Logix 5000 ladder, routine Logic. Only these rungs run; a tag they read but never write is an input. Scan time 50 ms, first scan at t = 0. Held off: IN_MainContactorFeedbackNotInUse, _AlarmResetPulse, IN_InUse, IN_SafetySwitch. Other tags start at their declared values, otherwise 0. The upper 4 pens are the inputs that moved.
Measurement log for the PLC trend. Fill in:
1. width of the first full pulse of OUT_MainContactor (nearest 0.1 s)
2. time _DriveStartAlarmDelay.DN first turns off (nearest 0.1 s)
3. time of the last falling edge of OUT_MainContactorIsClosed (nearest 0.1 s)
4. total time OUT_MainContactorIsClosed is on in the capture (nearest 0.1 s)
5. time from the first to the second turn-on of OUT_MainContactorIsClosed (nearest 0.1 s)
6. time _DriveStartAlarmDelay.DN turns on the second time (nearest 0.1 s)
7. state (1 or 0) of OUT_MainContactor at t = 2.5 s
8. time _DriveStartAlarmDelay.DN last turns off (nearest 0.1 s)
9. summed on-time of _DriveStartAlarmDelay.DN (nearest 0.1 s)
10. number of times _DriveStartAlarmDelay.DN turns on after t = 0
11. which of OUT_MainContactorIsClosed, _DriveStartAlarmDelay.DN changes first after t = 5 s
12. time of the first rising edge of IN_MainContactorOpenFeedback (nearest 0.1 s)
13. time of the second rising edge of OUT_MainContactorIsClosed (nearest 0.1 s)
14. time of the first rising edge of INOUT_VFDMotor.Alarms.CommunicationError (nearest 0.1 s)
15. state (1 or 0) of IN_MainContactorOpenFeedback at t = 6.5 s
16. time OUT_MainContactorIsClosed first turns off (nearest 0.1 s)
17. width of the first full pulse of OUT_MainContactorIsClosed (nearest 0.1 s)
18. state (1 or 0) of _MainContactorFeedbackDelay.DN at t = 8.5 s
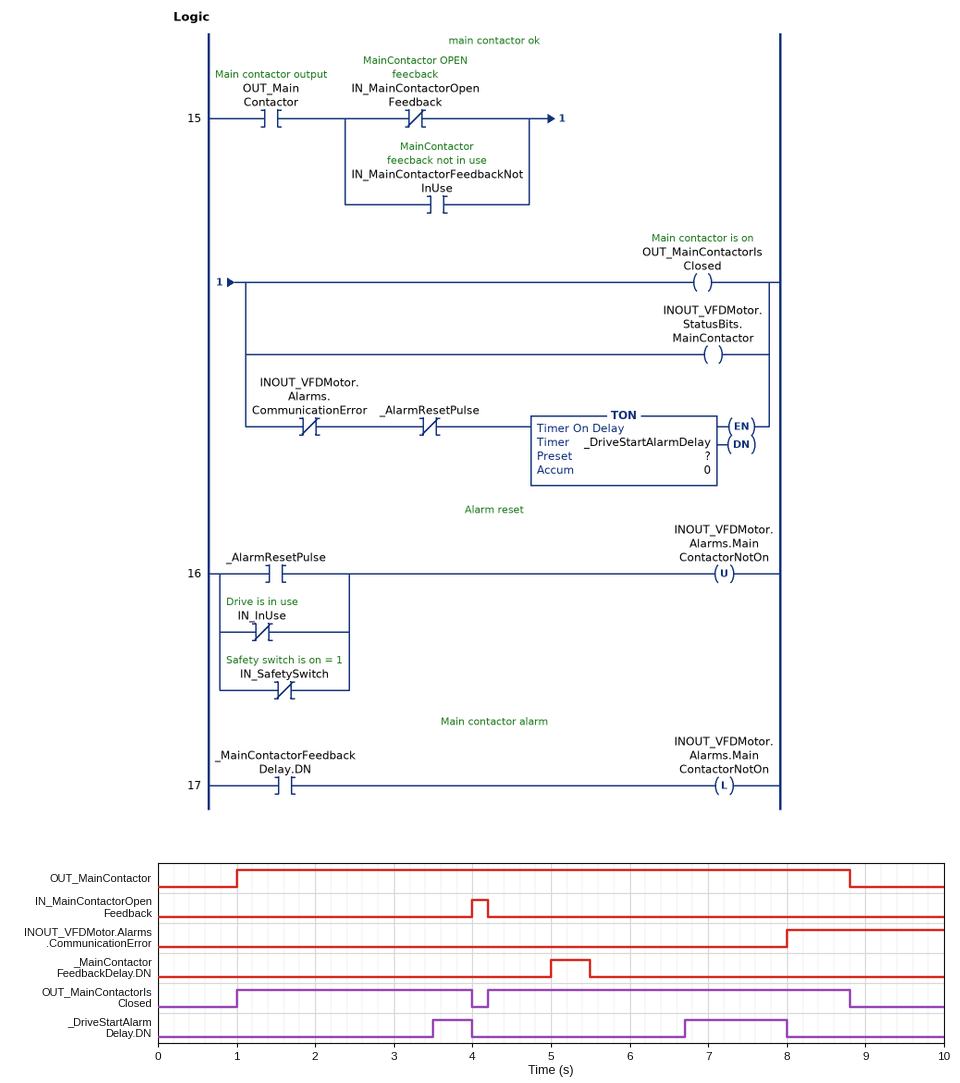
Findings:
7.8 s
4.0 s
8.8 s
7.6 s
3.2 s
6.7 s
1
8.0 s
1.8 s
2
_DriveStartAlarmDelay.DN
4.0 s
4.2 s
8.0 s
0
4.0 s
3.0 s
0
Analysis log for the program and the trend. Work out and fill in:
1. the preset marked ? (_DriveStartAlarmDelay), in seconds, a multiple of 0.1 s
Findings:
2.5 s
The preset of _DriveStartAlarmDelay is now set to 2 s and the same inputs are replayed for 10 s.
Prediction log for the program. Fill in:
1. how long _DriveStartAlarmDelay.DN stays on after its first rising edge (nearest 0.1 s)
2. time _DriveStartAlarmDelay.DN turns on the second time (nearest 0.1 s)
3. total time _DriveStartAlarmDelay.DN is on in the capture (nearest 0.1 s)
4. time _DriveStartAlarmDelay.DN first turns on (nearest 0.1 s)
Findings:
1.0 s
6.2 s
2.8 s
3.0 s
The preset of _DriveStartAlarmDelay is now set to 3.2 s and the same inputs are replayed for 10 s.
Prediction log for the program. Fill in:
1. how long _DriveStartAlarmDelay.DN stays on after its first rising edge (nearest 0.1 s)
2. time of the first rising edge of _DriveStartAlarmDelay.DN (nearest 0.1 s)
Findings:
0.6 s
7.4 s
